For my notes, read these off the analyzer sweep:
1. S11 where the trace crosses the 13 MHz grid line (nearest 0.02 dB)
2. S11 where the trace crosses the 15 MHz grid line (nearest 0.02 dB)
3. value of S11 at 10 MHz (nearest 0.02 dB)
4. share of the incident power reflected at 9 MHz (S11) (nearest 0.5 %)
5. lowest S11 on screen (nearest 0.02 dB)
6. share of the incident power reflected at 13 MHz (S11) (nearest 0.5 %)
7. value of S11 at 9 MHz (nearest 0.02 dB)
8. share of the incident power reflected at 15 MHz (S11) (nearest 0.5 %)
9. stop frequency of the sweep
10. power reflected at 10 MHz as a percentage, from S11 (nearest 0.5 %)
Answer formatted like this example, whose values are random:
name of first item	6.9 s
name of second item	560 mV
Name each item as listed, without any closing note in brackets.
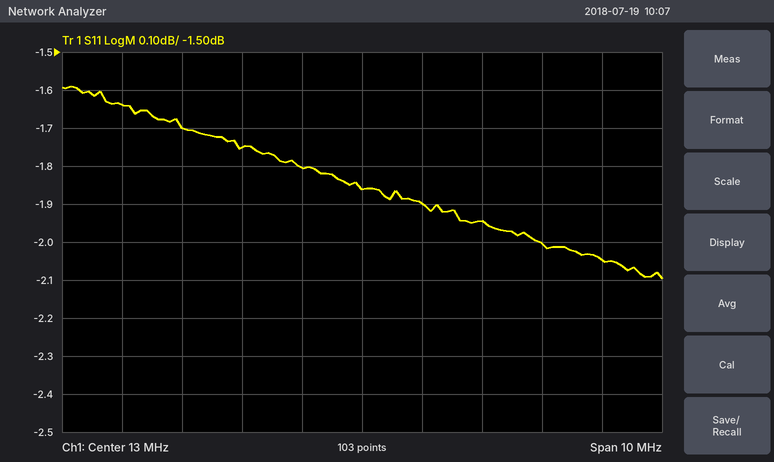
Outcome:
S11 where the trace crosses the 13 MHz grid line	-1.86 dB
S11 where the trace crosses the 15 MHz grid line	-1.94 dB
value of S11 at 10 MHz	-1.70 dB
share of the incident power reflected at 9 MHz (S11)	68.5 %
lowest S11 on screen	-2.10 dB
share of the incident power reflected at 13 MHz (S11)	65.0 %
value of S11 at 9 MHz	-1.64 dB
share of the incident power reflected at 15 MHz (S11)	64.0 %
stop frequency of the sweep	18 MHz
power reflected at 10 MHz as a percentage, from S11	67.5 %
